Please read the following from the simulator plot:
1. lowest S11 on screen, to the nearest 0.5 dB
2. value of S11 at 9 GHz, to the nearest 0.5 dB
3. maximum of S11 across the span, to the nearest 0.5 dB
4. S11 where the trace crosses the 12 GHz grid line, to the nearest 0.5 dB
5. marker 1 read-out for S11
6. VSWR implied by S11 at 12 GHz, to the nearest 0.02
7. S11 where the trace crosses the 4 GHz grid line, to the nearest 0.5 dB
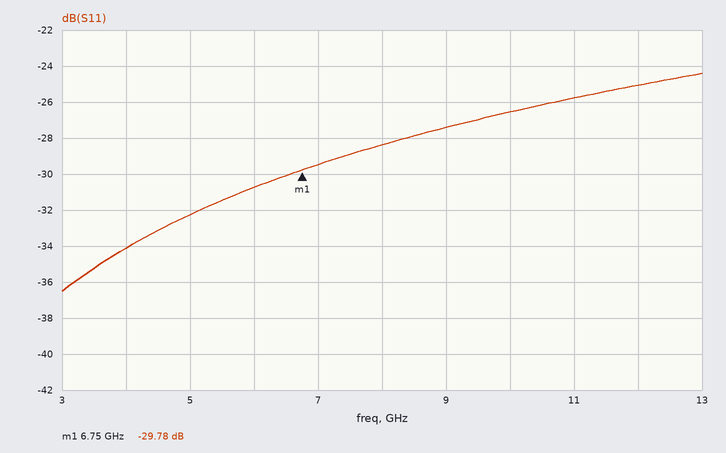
-36.5 dB
-27.5 dB
-24.5 dB
-25.0 dB
-29.78 dB
1.12
-34.0 dB
